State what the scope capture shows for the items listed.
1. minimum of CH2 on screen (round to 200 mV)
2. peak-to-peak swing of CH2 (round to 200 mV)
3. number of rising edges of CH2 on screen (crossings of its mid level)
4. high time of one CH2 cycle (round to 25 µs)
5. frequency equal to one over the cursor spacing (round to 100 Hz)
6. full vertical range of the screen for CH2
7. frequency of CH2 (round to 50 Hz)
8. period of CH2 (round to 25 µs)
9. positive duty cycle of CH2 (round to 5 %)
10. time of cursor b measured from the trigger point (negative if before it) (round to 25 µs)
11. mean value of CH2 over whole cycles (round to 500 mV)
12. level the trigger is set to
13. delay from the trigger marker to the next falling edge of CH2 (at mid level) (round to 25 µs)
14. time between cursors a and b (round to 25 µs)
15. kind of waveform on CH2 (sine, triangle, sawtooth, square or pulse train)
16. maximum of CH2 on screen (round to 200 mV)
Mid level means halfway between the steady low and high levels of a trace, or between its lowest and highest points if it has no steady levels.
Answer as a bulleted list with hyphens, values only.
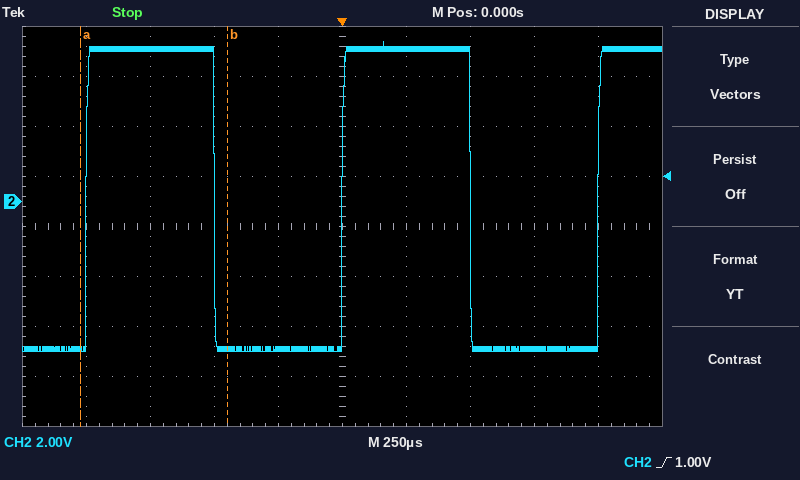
- -6.0 V
- 12.4 V
- 3
- 500 µs
- 1.7 kHz
- 16 V
- 1.00 kHz
- 1.000 ms
- 50 %
- -450 µs
- 0.0 V
- 1.00 V
- 500 µs
- 575 µs
- square
- 6.4 V
